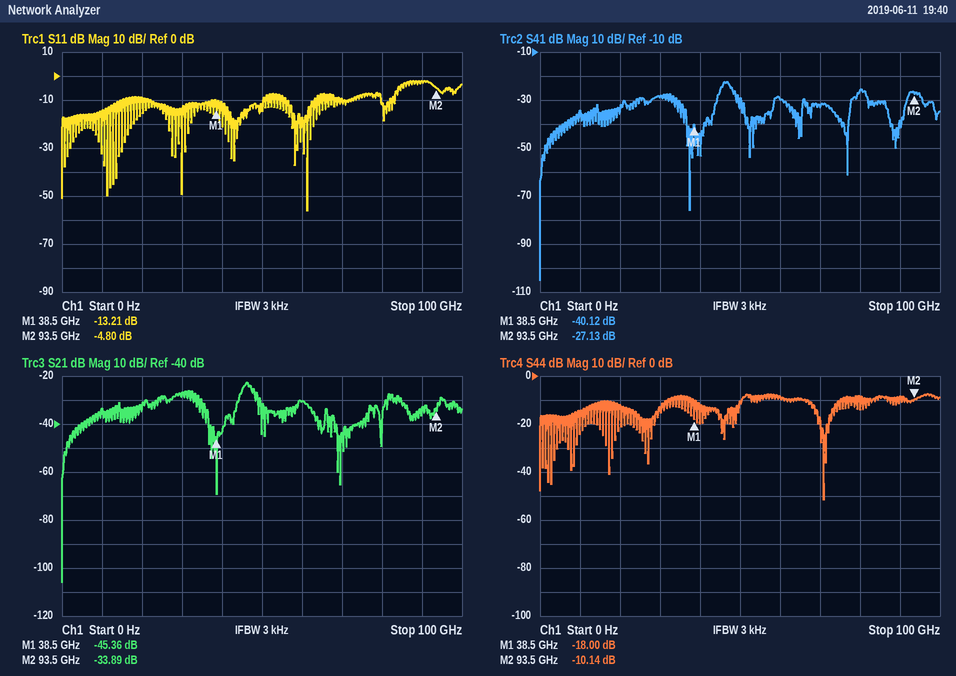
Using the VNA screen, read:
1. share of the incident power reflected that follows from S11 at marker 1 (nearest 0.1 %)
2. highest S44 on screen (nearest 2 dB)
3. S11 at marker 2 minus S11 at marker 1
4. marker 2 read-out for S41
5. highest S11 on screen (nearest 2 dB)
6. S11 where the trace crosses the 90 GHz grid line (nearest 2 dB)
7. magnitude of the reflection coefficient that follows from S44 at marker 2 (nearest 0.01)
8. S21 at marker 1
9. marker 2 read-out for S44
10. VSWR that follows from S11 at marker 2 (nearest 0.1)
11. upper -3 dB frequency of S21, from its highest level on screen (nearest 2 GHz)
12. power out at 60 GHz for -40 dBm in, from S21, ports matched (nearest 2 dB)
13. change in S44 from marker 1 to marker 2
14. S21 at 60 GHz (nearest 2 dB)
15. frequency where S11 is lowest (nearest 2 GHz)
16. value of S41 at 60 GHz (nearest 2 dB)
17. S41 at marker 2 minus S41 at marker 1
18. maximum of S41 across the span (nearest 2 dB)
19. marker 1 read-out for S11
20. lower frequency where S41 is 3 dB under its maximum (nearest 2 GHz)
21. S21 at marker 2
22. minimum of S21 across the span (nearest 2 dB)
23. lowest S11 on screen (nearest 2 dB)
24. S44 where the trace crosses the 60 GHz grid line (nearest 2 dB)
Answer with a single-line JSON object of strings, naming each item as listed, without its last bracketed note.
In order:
{"share of the incident power reflected that follows from S11 at marker 1": "4.8 %", "highest S44 on screen": "-8 dB", "S11 at marker 2 minus S11 at marker 1": "8.41 dB", "marker 2 read-out for S41": "-27.13 dB", "highest S11 on screen": "-2 dB", "S11 where the trace crosses the 90 GHz grid line": "-2 dB", "magnitude of the reflection coefficient that follows from S44 at marker 2": "0.31", "S21 at marker 1": "-45.36 dB", "marker 2 read-out for S44": "-10.14 dB", "VSWR that follows from S11 at marker 2": "3.7", "upper -3 dB frequency of S21, from its highest level on screen": "48 GHz", "power out at 60 GHz for -40 dBm in, from S21, ports matched": "-70 dBm", "change in S44 from marker 1 to marker 2": "7.86 dB", "S21 at 60 GHz": "-30 dB", "frequency where S11 is lowest": "62 GHz", "value of S41 at 60 GHz": "-30 dB", "S41 at marker 2 minus S41 at marker 1": "12.99 dB", "maximum of S41 across the span": "-22 dB", "marker 1 read-out for S11": "-13.21 dB", "lower frequency where S41 is 3 dB under its maximum": "46 GHz", "S21 at marker 2": "-33.89 dB", "minimum of S21 across the span": "-106 dB", "lowest S11 on screen": "-56 dB", "S44 where the trace crosses the 60 GHz grid line": "-8 dB"}
